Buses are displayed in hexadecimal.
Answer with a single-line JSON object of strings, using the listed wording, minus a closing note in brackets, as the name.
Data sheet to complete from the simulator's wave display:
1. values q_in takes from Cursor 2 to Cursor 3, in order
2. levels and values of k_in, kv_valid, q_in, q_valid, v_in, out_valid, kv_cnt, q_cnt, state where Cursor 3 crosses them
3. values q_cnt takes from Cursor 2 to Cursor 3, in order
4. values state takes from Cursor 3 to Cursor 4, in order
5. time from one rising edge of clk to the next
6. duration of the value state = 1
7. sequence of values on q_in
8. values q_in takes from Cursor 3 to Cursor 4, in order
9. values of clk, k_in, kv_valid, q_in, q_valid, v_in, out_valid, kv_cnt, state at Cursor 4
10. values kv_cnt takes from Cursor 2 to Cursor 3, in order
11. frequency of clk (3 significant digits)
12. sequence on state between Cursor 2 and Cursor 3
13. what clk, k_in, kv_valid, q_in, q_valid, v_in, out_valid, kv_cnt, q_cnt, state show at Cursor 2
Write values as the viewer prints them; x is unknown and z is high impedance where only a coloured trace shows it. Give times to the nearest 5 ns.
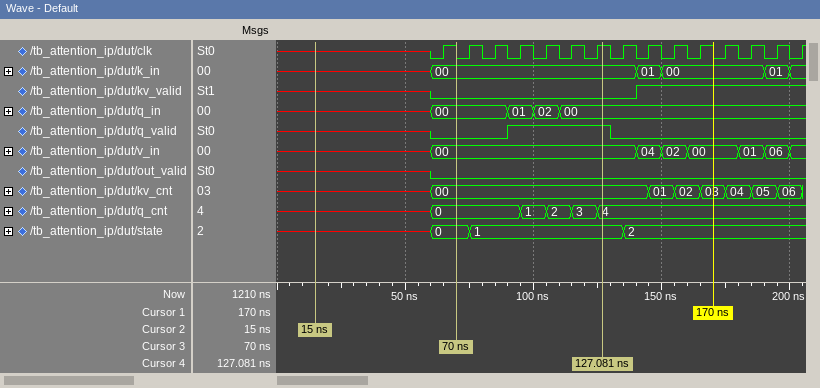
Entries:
{"values q_in takes from Cursor 2 to Cursor 3, in order": "x, 00", "levels and values of k_in, kv_valid, q_in, q_valid, v_in, out_valid, kv_cnt, q_cnt, state where Cursor 3 crosses them": "k_in=00, kv_valid=0, q_in=00, q_valid=0, v_in=00, out_valid=0, kv_cnt=00, q_cnt=0, state=0", "values q_cnt takes from Cursor 2 to Cursor 3, in order": "x, 0", "values state takes from Cursor 3 to Cursor 4, in order": "0, 1", "time from one rising edge of clk to the next": "10 ns", "duration of the value state = 1": "60 ns", "sequence of values on q_in": "x, 00, 01, 02, 00", "values q_in takes from Cursor 3 to Cursor 4, in order": "00, 01, 02, 00", "values of clk, k_in, kv_valid, q_in, q_valid, v_in, out_valid, kv_cnt, state at Cursor 4": "clk=1, k_in=00, kv_valid=0, q_in=00, q_valid=1, v_in=00, out_valid=0, kv_cnt=00, state=1", "values kv_cnt takes from Cursor 2 to Cursor 3, in order": "x, 00", "frequency of clk": "100 MHz", "sequence on state between Cursor 2 and Cursor 3": "x, 0", "what clk, k_in, kv_valid, q_in, q_valid, v_in, out_valid, kv_cnt, q_cnt, state show at Cursor 2": "clk=x, k_in=x, kv_valid=x, q_in=x, q_valid=x, v_in=x, out_valid=x, kv_cnt=x, q_cnt=x, state=x"}
